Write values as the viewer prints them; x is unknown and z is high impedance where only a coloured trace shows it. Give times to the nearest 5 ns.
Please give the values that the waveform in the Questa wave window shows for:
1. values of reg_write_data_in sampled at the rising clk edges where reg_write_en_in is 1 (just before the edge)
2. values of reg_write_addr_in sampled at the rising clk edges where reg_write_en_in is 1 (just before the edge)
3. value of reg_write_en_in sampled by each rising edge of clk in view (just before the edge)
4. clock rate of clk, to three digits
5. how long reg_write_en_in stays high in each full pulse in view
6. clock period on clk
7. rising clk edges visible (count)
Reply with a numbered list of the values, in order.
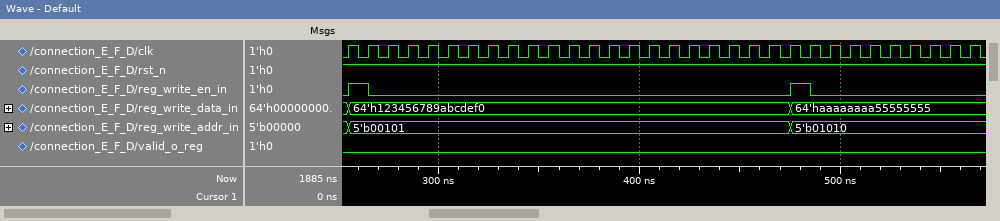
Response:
1. 64'h123456789abcdef0, 64'haaaaaaaa55555555
2. 5'b00101, 5'b01010
3. 0 1 0 0 0 0 0 0 0 0 0 0 0 0 0 0 0 0 0 0 0 0 0 1 0 0 0 0 0 0 0 0
4. 100 MHz
5. 10 ns, 10 ns
6. 10 ns
7. 32
